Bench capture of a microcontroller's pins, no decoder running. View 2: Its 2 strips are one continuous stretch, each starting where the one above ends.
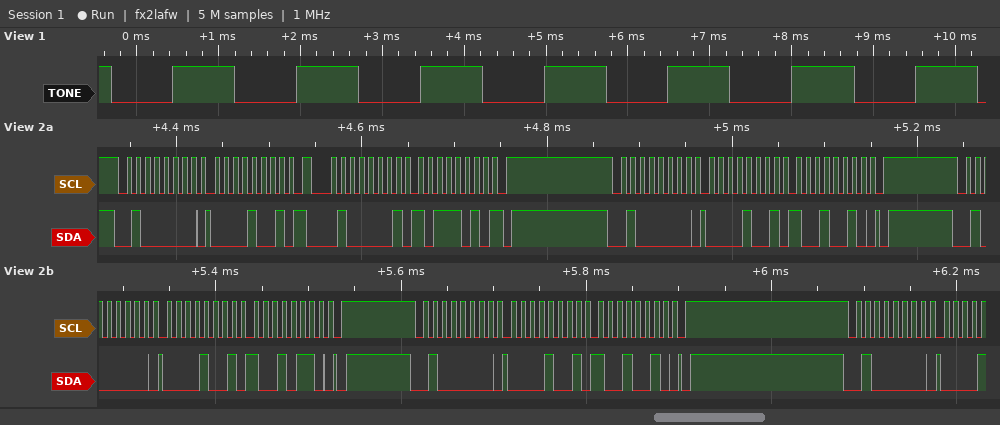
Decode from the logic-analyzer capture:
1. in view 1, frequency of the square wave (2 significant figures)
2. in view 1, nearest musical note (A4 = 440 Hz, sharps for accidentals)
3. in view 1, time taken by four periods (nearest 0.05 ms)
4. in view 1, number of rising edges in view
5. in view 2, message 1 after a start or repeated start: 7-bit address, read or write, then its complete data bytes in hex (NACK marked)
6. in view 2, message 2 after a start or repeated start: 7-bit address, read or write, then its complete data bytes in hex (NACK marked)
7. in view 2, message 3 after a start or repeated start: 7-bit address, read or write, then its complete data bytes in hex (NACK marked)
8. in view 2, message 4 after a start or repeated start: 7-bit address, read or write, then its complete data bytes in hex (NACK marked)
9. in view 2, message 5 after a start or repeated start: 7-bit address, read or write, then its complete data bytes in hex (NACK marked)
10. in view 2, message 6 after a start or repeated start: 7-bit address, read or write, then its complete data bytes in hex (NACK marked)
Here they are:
660 Hz
E5
6.05 ms
7
0x20 write: 09
0x20 read: BA NACK
0x20 write: 09 92
0x20 write: 09 96
0x20 write: 09 92
0x20 write
